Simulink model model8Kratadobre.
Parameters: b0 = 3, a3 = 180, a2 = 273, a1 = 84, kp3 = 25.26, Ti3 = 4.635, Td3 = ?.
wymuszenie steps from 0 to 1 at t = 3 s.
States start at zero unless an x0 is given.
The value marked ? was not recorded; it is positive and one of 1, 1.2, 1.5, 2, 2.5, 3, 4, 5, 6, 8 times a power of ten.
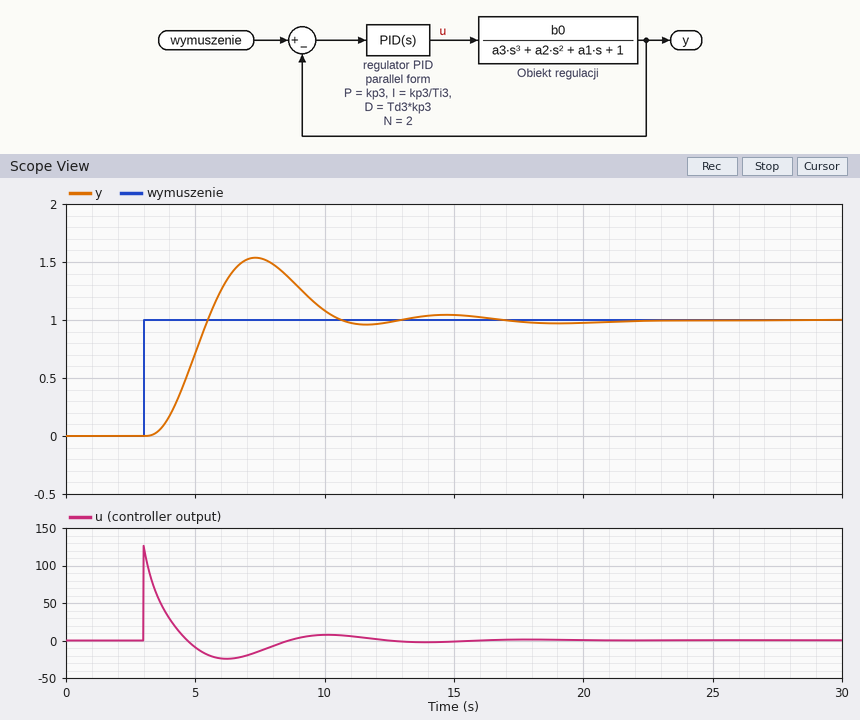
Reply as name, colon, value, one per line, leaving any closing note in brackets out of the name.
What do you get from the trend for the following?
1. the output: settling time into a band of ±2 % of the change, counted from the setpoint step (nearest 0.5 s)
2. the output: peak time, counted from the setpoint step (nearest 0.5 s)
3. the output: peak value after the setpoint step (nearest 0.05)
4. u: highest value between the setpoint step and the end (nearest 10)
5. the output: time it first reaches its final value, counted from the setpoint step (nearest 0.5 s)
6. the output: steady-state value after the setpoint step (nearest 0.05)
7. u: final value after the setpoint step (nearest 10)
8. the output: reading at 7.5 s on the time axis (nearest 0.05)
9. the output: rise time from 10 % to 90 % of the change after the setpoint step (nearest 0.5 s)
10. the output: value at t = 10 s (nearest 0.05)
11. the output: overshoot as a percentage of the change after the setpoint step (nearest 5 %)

the output: settling time into a band of ±2 % of the change, counted from the setpoint step: 17.5 s
the output: peak time, counted from the setpoint step: 4.5 s
the output: peak value after the setpoint step: 1.55
u: highest value between the setpoint step and the end: 130
the output: time it first reaches its final value, counted from the setpoint step: 2.5 s
the output: steady-state value after the setpoint step: 1.00
u: final value after the setpoint step: 0
the output: reading at 7.5 s on the time axis: 1.55
the output: rise time from 10 % to 90 % of the change after the setpoint step: 1.5 s
the output: value at t = 10 s: 1.10
the output: overshoot as a percentage of the change after the setpoint step: 55 %
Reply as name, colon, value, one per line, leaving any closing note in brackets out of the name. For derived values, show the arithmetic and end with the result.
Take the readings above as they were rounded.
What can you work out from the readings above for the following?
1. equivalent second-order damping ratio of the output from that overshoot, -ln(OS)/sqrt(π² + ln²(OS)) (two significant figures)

equivalent second-order damping ratio of the output from that overshoot, -ln(OS)/sqrt(π² + ln²(OS)): ln(0.55) = -0.598; 0.598 / sqrt(9.870 + 0.357) = 0.19
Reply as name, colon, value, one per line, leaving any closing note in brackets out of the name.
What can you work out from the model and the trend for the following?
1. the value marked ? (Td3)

the value marked ?: 2
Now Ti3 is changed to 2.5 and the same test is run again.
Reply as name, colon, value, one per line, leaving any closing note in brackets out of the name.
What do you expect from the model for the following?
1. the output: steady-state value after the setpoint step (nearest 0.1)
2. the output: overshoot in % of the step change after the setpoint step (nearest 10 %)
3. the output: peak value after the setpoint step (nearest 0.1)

the output: steady-state value after the setpoint step: 1.0
the output: overshoot in % of the step change after the setpoint step: 70 %
the output: peak value after the setpoint step: 1.7
